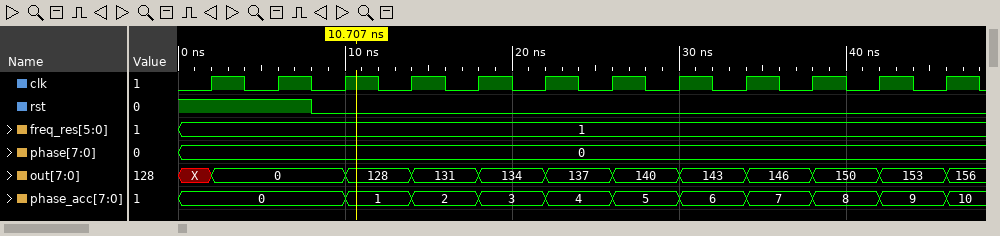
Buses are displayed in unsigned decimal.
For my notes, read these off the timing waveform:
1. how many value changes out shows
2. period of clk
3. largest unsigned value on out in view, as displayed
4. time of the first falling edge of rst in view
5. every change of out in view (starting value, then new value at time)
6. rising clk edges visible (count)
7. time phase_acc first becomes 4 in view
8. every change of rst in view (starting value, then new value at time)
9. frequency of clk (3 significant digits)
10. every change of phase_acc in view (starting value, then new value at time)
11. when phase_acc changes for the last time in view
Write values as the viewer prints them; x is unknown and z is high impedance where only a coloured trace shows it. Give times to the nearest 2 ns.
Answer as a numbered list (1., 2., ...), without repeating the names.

1. 11
2. 4 ns
3. 156
4. 8 ns
5. X, 0 at 2 ns, 128 at 10 ns, 131 at 14 ns, 134 at 18 ns, 137 at 22 ns, 140 at 26 ns, 143 at 30 ns, 146 at 34 ns, 150 at 38 ns, 153 at 42 ns, 156 at 46 ns
6. 12
7. 22 ns
8. 1, 0 at 8 ns
9. 250 MHz
10. 0, 1 at 10 ns, 2 at 14 ns, 3 at 18 ns, 4 at 22 ns, 5 at 26 ns, 6 at 30 ns, 7 at 34 ns, 8 at 38 ns, 9 at 42 ns, 10 at 46 ns
11. 46 ns
